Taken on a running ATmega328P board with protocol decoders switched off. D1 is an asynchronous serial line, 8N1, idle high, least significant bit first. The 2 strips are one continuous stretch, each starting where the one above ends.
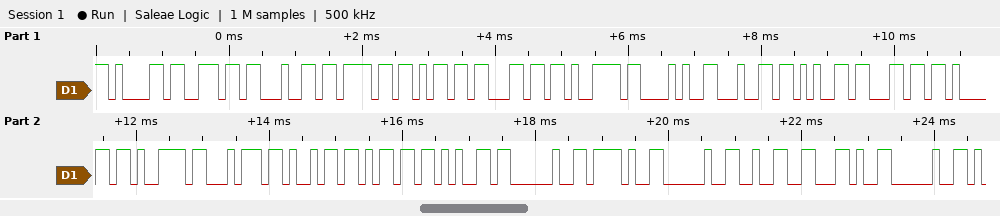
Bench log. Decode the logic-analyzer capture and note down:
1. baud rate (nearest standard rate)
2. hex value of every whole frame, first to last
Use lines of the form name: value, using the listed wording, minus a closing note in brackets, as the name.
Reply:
baud rate: 9600 baud
hex value of every whole frame, first to last: 0x61 0x6E 0x64 0x6F 0x6D 0x6C 0x79 0x28 0x64 0x65 0x6C 0x61 0x79 0x74 0x69 0x6D 0x65 0x20 0x2F 0x20 0x32 0x2C 0x20
